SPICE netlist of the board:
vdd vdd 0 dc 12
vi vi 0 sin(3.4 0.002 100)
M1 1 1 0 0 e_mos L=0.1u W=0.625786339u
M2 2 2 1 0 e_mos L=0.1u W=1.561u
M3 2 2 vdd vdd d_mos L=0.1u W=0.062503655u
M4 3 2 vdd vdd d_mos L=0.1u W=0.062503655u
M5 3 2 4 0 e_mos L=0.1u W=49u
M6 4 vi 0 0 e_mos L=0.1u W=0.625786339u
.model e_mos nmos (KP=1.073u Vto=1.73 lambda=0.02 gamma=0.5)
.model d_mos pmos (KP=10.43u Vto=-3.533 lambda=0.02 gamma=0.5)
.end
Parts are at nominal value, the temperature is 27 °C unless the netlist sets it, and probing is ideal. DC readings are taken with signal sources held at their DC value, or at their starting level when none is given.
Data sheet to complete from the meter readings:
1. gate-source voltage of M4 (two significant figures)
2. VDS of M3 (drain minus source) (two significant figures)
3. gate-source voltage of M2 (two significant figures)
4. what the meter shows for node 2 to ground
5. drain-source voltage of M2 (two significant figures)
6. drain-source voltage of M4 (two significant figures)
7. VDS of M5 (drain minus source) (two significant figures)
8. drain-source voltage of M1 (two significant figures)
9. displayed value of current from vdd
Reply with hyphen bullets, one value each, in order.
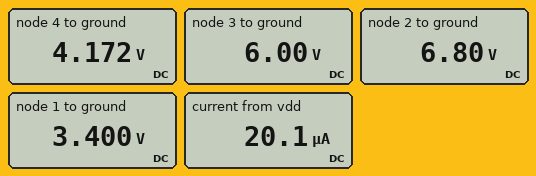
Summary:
- -5.2 V
- -5.2 V
- 3.4 V
- 6.80 V
- 3.4 V
- -6.0 V
- 1.8 V
- 3.4 V
- 20.1 µA
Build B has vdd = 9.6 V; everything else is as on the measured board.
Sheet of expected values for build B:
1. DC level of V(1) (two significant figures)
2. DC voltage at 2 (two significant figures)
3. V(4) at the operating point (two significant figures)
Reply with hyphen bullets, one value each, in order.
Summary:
- 2.5 V
- 5.3 V
- 240 mV
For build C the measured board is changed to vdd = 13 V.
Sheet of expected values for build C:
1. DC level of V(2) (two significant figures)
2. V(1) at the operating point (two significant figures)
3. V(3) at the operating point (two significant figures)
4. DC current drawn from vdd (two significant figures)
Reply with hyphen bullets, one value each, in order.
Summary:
- 7.4 V
- 3.8 V
- 12 V
- 25 µA
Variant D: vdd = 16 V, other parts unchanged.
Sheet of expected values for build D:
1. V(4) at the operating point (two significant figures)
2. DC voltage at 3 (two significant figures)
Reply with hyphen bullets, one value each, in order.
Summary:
- 6.5 V
- 15 V
